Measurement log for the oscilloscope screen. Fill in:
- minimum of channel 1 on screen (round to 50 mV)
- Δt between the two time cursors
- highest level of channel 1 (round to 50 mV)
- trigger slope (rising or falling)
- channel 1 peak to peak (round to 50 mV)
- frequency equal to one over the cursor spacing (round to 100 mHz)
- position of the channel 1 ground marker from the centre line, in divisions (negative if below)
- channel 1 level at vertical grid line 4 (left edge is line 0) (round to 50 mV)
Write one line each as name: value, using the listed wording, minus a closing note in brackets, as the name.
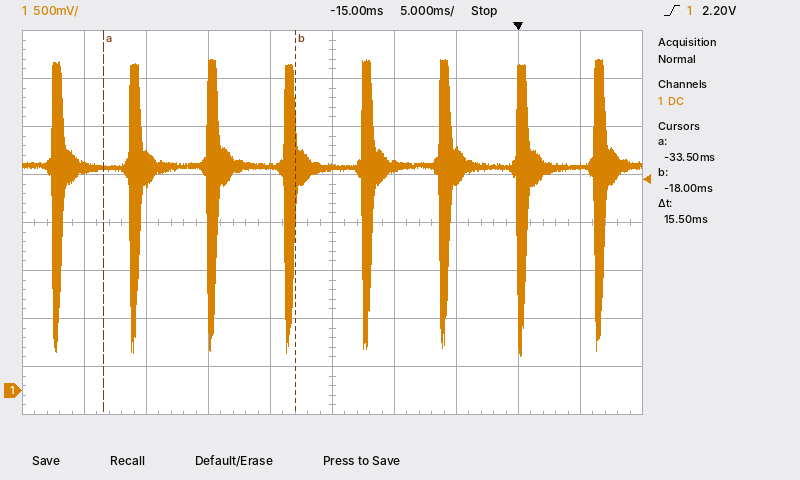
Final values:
minimum of channel 1 on screen: 350 mV
Δt between the two time cursors: 15.5 ms
highest level of channel 1: 3.45 V
trigger slope: rising
channel 1 peak to peak: 3.10 V
frequency equal to one over the cursor spacing: 64.5 Hz
position of the channel 1 ground marker from the centre line, in divisions: -3.5 div
channel 1 level at vertical grid line 4 (left edge is line 0): 2.35 V
